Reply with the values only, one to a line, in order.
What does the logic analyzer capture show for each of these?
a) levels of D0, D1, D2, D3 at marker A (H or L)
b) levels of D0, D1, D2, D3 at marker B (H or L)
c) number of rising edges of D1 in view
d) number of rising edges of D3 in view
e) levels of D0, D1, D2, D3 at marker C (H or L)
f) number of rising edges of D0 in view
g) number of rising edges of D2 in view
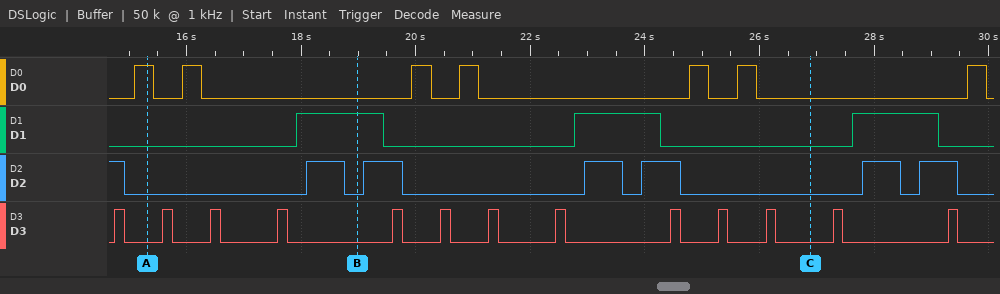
D0=H, D1=L, D2=L, D3=L
D0=L, D1=H, D2=L, D3=L
3
13
D0=L, D1=L, D2=L, D3=L
7
6
